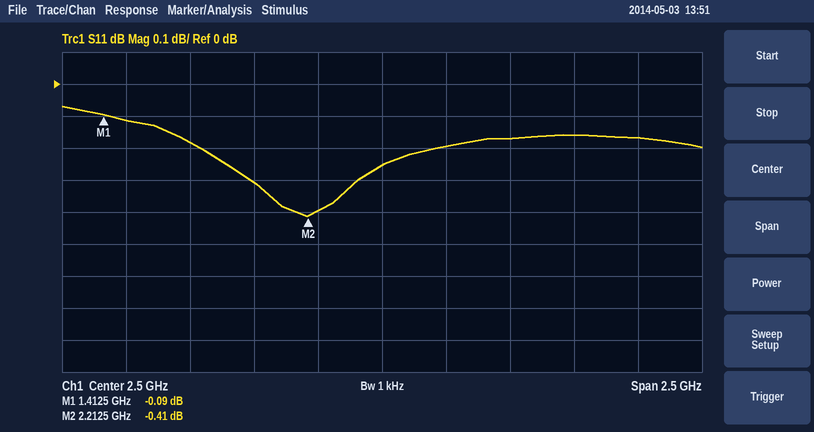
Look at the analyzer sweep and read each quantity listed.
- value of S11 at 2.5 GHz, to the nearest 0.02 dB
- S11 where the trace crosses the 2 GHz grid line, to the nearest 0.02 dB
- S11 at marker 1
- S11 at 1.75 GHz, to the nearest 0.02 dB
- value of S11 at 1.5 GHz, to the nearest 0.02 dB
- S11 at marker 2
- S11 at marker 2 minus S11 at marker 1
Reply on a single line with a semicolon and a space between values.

-0.26 dB; -0.30 dB; -0.09 dB; -0.18 dB; -0.12 dB; -0.41 dB; -0.32 dB
